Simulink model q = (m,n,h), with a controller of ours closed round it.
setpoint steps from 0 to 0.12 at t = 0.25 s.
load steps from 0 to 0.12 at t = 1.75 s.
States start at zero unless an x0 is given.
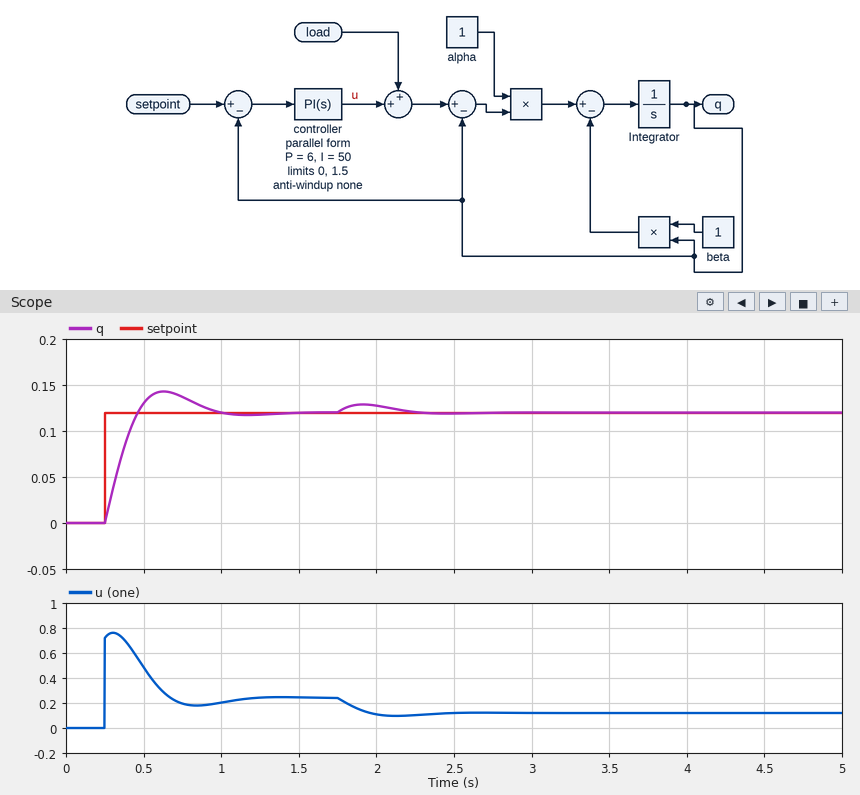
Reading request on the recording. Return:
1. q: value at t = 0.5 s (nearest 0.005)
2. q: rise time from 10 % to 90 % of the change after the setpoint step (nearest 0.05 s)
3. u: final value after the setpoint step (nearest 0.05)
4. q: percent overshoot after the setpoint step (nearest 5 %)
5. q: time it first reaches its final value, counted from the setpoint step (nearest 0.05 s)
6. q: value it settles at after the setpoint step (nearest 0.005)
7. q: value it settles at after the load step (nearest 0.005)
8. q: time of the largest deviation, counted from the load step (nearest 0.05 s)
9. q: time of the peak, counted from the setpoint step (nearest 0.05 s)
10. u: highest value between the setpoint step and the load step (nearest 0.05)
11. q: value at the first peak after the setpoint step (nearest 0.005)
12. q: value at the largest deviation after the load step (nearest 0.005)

0.130
0.15 s
0.25
20 %
0.20 s
0.120
0.120
0.15 s
0.40 s
0.75
0.145
0.130
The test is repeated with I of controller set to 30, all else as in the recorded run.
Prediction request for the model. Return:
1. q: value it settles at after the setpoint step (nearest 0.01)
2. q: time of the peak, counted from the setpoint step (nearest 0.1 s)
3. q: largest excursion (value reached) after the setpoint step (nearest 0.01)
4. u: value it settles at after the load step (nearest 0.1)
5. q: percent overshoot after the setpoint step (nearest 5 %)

0.12
0.5 s
0.13
0.1
10 %
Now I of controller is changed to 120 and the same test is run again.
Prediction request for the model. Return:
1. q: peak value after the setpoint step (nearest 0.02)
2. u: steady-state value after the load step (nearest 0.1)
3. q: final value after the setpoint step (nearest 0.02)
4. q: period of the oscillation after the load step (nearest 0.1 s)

0.16
0.1
0.12
0.6 s
